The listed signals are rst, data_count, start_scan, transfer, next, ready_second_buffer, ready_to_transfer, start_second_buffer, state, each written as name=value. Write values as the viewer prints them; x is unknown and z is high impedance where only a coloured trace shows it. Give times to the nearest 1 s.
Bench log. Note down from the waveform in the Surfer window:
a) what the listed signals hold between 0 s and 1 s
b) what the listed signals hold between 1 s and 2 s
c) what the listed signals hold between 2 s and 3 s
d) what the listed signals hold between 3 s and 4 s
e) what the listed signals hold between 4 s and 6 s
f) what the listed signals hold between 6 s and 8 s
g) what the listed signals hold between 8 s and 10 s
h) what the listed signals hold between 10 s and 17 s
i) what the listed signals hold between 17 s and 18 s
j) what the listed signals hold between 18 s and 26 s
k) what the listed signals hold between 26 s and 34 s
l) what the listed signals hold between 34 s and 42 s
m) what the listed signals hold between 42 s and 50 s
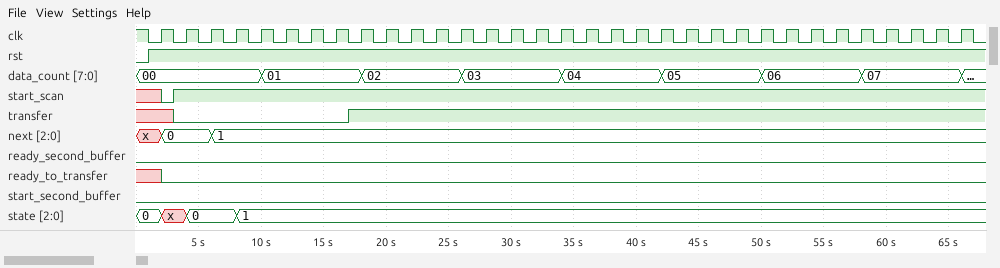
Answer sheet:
rst=0, data_count=00, start_scan=x, transfer=x, next=x, ready_second_buffer=0, ready_to_transfer=x, start_second_buffer=0, state=0
rst=1, data_count=00, start_scan=x, transfer=x, next=x, ready_second_buffer=0, ready_to_transfer=x, start_second_buffer=0, state=0
rst=1, data_count=00, start_scan=0, transfer=x, next=0, ready_second_buffer=0, ready_to_transfer=0, start_second_buffer=0, state=x
rst=1, data_count=00, start_scan=1, transfer=0, next=0, ready_second_buffer=0, ready_to_transfer=0, start_second_buffer=0, state=x
rst=1, data_count=00, start_scan=1, transfer=0, next=0, ready_second_buffer=0, ready_to_transfer=0, start_second_buffer=0, state=0
rst=1, data_count=00, start_scan=1, transfer=0, next=1, ready_second_buffer=0, ready_to_transfer=0, start_second_buffer=0, state=0
rst=1, data_count=00, start_scan=1, transfer=0, next=1, ready_second_buffer=0, ready_to_transfer=0, start_second_buffer=0, state=1
rst=1, data_count=01, start_scan=1, transfer=0, next=1, ready_second_buffer=0, ready_to_transfer=0, start_second_buffer=0, state=1
rst=1, data_count=01, start_scan=1, transfer=1, next=1, ready_second_buffer=0, ready_to_transfer=0, start_second_buffer=0, state=1
rst=1, data_count=02, start_scan=1, transfer=1, next=1, ready_second_buffer=0, ready_to_transfer=0, start_second_buffer=0, state=1
rst=1, data_count=03, start_scan=1, transfer=1, next=1, ready_second_buffer=0, ready_to_transfer=0, start_second_buffer=0, state=1
rst=1, data_count=04, start_scan=1, transfer=1, next=1, ready_second_buffer=0, ready_to_transfer=0, start_second_buffer=0, state=1
rst=1, data_count=05, start_scan=1, transfer=1, next=1, ready_second_buffer=0, ready_to_transfer=0, start_second_buffer=0, state=1
